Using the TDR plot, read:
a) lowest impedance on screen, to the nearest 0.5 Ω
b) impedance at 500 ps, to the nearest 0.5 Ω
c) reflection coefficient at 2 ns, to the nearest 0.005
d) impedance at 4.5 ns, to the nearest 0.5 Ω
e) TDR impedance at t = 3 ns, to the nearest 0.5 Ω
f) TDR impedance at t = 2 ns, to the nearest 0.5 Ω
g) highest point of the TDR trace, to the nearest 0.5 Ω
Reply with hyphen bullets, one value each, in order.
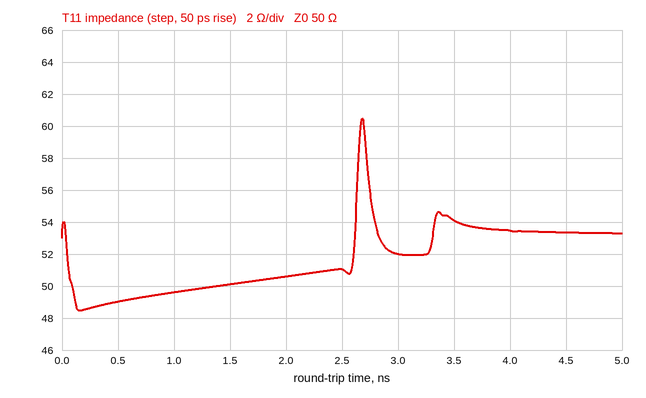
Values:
- 48.5 Ω
- 49.0 Ω
- +0.005
- 53.5 Ω
- 52.0 Ω
- 50.5 Ω
- 60.5 Ω
